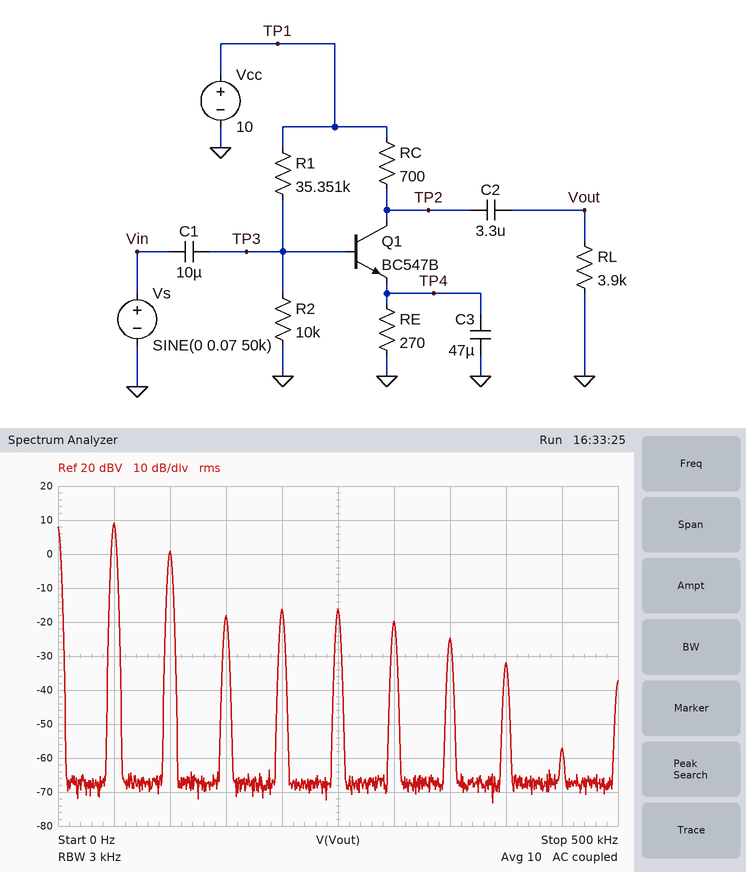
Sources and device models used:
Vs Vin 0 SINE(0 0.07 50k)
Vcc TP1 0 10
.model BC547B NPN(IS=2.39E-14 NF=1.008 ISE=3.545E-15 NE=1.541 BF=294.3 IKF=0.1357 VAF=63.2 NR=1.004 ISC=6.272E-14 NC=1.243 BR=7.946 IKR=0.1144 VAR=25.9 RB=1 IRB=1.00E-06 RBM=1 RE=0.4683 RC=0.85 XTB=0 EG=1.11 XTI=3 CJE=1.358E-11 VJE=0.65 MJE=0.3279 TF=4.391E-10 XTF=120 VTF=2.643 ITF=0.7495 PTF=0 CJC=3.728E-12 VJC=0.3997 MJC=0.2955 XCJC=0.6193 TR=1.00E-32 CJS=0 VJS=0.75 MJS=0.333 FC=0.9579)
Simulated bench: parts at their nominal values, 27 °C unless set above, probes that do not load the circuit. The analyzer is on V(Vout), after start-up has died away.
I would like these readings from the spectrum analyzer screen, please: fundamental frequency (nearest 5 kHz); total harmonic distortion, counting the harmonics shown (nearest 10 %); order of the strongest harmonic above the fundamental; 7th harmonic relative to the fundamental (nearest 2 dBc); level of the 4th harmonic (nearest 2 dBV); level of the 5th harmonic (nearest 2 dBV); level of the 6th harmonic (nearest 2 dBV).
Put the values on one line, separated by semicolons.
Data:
50 kHz; 40 %; 2; -34 dBc; -16 dBV; -16 dBV; -20 dBV
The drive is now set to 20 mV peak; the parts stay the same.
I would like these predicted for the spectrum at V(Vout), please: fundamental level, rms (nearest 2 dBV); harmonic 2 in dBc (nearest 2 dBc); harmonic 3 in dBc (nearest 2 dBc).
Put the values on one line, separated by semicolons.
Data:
2 dBV; -18 dBc; -42 dBc
